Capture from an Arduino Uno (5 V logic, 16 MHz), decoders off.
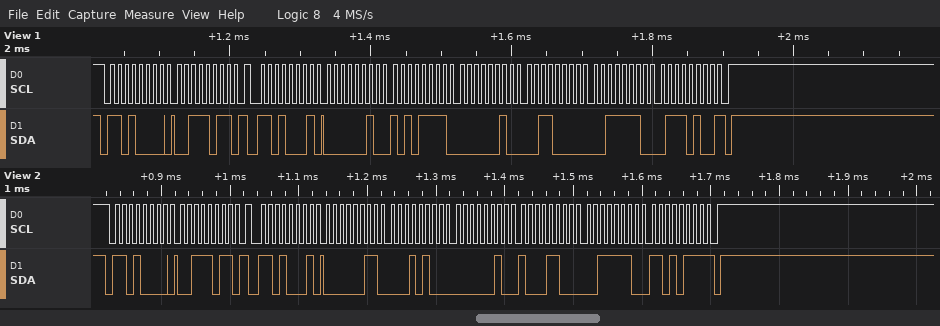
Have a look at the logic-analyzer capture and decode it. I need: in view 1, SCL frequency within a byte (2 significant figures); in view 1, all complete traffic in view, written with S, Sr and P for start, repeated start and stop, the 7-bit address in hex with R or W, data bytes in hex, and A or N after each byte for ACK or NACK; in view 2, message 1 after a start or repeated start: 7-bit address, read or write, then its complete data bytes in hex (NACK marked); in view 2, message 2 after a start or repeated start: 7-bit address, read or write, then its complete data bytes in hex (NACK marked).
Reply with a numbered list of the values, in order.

1. 100 kHz
2. S 68W A 3B A Sr 68R A 02 A AF A 02 A 30 A 3E A 74 N P
3. 0x68 write: 3B
4. 0x68 read: 03 14 02 8C 3E D7 NACK
